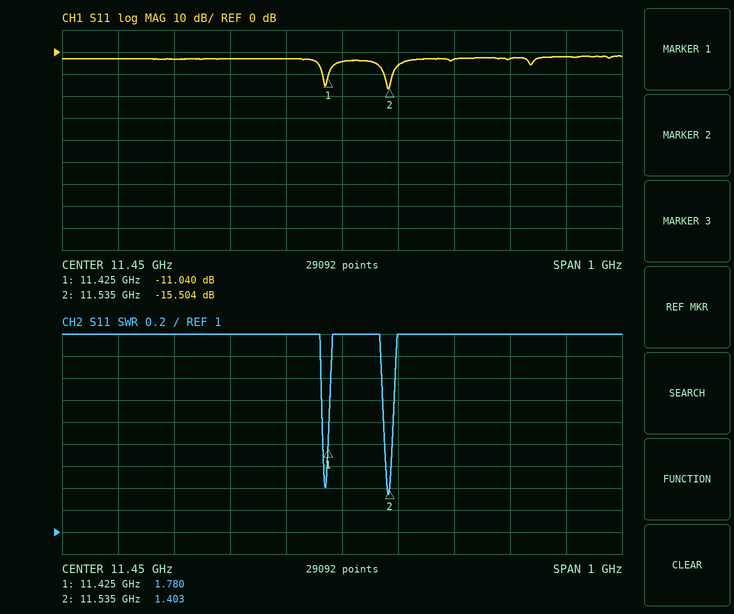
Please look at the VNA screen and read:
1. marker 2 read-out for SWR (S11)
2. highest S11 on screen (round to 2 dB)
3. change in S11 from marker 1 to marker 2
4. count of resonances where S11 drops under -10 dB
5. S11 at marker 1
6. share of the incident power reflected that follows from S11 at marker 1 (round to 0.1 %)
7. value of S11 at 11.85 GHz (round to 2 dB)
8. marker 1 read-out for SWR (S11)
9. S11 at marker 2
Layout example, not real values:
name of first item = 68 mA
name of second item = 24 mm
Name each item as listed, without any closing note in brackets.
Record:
marker 2 read-out for SWR = 1.403
highest S11 on screen = -2 dB
change in S11 from marker 1 to marker 2 = -4.464 dB
count of resonances where S11 drops under -10 dB = 2
S11 at marker 1 = -11.040 dB
share of the incident power reflected that follows from S11 at marker 1 = 7.9 %
value of S11 at 11.85 GHz = -2 dB
marker 1 read-out for SWR = 1.780
S11 at marker 2 = -15.504 dB
